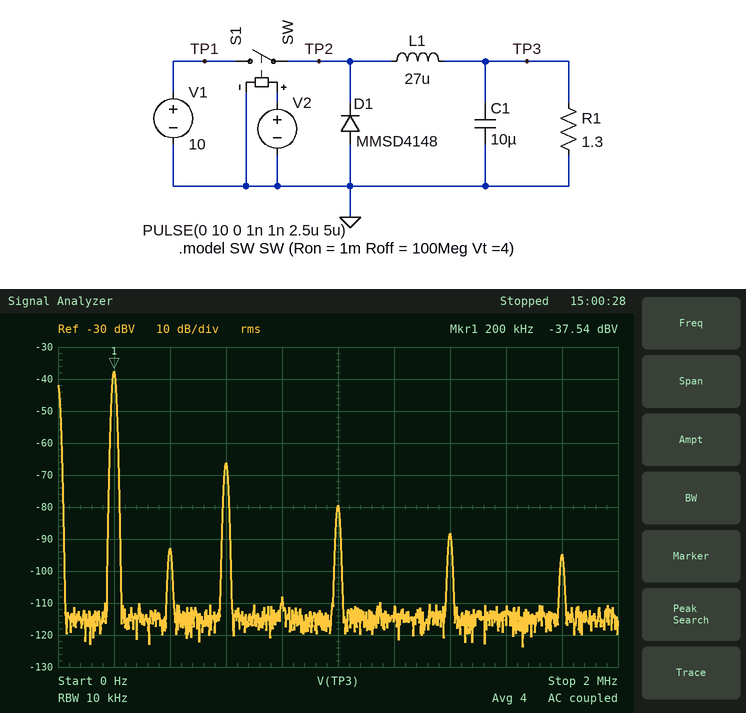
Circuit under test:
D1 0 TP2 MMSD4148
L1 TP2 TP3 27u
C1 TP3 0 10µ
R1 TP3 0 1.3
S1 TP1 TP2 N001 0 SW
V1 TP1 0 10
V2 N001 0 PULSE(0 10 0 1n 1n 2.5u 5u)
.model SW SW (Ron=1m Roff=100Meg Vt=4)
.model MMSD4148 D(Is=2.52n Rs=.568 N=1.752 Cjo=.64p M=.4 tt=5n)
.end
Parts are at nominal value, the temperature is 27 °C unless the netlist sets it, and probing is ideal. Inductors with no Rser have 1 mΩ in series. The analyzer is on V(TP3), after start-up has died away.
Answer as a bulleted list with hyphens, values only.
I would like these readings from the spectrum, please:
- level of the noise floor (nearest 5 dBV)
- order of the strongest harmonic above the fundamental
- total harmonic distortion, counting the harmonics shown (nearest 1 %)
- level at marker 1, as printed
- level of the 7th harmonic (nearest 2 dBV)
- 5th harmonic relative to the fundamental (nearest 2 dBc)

- -115 dBV
- 3
- 4 %
- -37.54 dBV
- -88 dBV
- -42 dBc
